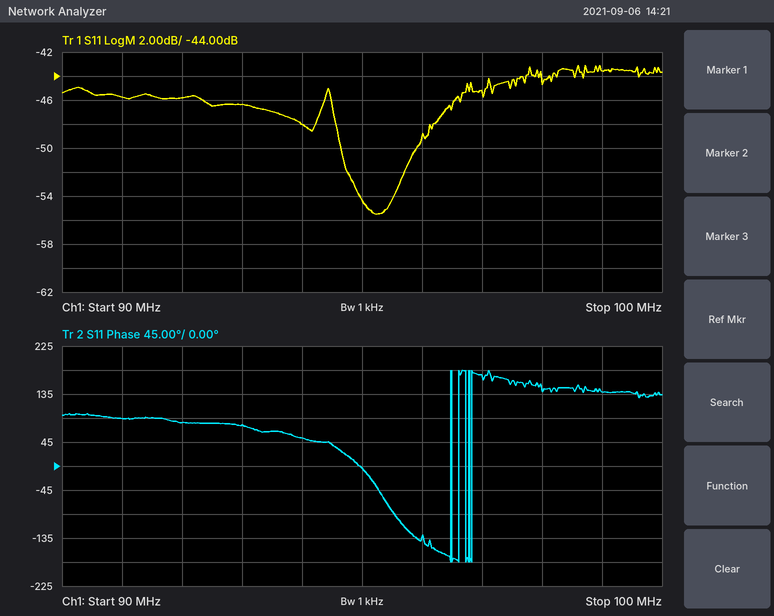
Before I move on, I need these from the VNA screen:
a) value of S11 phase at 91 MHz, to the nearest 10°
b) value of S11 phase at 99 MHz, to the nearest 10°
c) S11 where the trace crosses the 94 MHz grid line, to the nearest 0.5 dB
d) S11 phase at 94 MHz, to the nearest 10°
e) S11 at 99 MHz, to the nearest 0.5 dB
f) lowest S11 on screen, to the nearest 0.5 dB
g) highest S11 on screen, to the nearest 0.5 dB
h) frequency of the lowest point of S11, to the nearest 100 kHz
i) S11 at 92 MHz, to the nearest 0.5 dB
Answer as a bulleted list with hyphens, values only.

- 90°
- 140°
- -48.0 dB
- 50°
- -43.5 dB
- -55.5 dB
- -43.0 dB
- 95.2 MHz
- -46.0 dB
